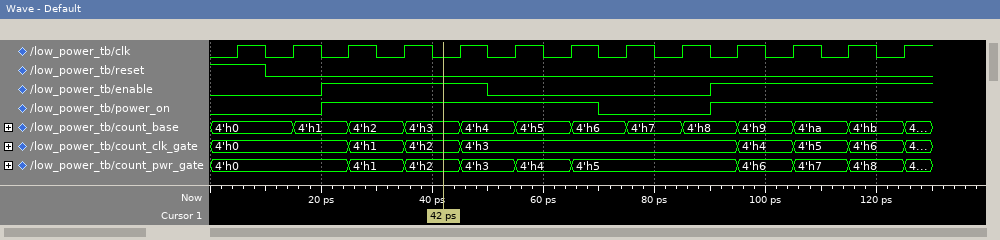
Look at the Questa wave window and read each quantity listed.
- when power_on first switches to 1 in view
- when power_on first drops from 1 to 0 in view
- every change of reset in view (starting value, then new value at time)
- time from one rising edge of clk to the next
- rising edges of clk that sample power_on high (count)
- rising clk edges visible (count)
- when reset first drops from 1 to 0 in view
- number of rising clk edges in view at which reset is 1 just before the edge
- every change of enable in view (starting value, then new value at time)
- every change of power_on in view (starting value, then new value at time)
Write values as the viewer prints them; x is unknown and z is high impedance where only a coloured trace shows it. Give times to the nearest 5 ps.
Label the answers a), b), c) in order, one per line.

a) 20 ps
b) 70 ps
c) 1, 0 at 10 ps
d) 10 ps
e) 9
f) 13
g) 10 ps
h) 1
i) 0, 1 at 20 ps, 0 at 50 ps, 1 at 90 ps
j) 0, 1 at 20 ps, 0 at 70 ps, 1 at 90 ps
